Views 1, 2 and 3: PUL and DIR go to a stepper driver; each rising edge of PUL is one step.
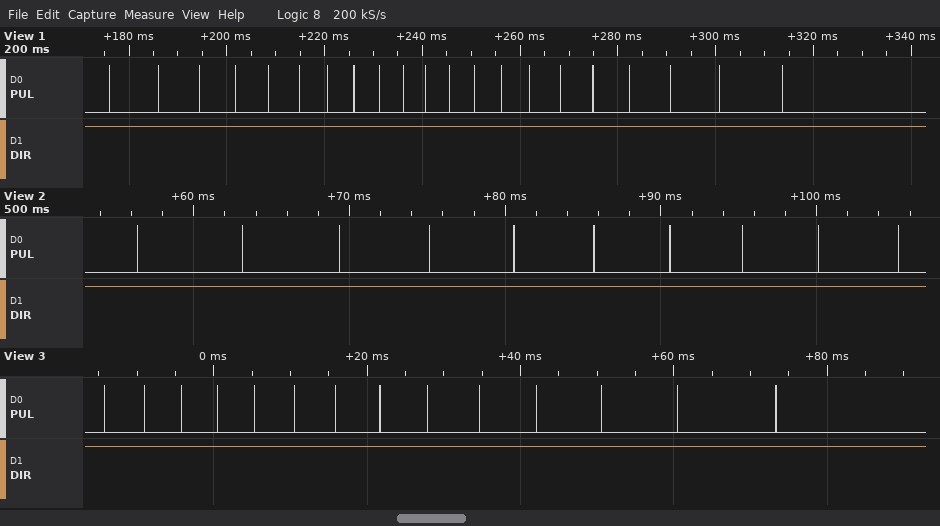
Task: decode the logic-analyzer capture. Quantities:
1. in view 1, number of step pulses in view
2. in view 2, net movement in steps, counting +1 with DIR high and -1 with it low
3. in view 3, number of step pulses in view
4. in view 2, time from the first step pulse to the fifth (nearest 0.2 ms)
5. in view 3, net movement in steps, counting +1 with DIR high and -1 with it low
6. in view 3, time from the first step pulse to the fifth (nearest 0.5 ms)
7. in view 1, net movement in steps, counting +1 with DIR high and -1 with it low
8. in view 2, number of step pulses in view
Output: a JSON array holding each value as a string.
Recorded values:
["21", "+10", "14", "24.2 ms", "+14", "19.5 ms", "+21", "10"]
